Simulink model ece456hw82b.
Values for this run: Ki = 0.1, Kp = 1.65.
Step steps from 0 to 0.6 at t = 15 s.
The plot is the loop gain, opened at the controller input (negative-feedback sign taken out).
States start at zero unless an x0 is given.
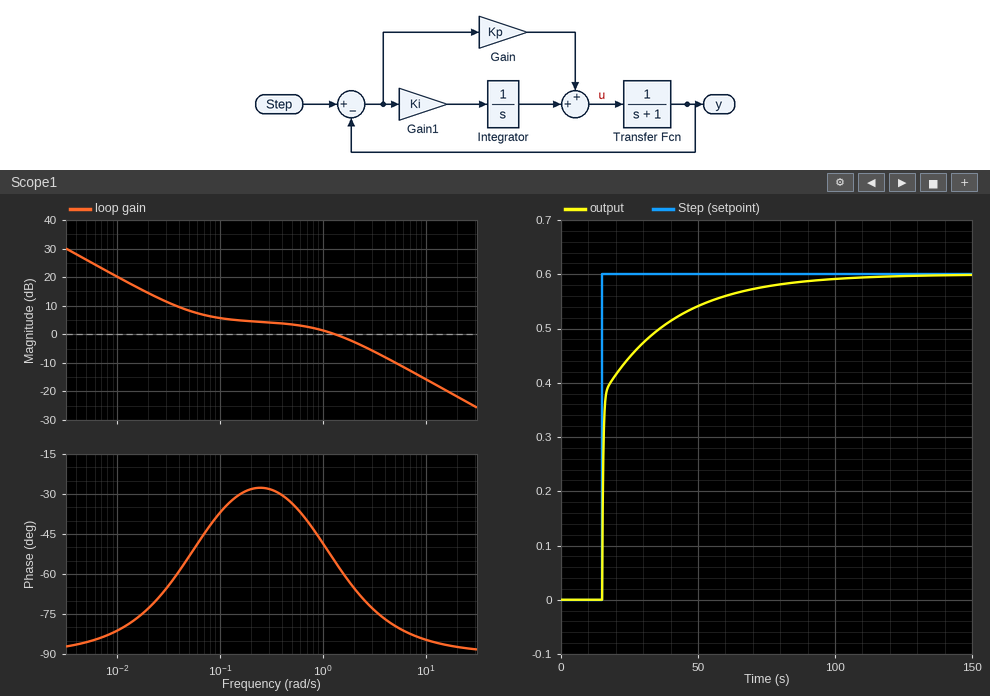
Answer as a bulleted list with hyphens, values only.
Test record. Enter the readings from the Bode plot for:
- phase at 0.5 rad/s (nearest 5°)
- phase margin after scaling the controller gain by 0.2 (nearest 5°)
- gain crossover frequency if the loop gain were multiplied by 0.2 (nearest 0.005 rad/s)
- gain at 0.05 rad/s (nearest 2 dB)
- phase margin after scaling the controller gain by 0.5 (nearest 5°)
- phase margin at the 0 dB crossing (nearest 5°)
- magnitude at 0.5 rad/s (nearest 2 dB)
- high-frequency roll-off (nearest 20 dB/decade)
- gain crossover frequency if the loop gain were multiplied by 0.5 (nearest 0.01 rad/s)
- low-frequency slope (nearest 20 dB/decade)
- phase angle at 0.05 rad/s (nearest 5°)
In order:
- -35°
- 110°
- 0.020 rad/s
- 8 dB
- 140°
- 125°
- 4 dB
- -20 dB/decade
- 0.09 rad/s
- -20 dB/decade
- -55°
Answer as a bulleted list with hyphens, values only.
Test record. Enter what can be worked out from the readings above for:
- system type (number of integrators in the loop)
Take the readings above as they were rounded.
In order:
- 1
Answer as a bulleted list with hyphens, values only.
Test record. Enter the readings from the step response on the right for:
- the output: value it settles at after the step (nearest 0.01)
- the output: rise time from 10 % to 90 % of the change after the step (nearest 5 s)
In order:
- 0.60
- 35 s
